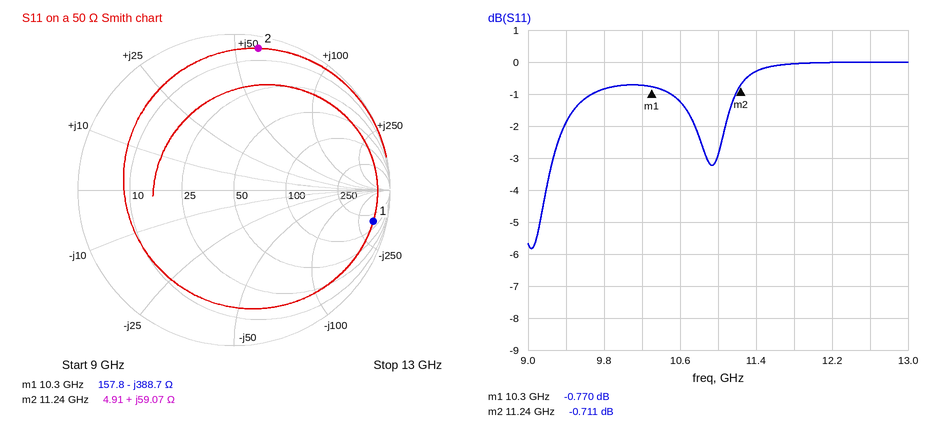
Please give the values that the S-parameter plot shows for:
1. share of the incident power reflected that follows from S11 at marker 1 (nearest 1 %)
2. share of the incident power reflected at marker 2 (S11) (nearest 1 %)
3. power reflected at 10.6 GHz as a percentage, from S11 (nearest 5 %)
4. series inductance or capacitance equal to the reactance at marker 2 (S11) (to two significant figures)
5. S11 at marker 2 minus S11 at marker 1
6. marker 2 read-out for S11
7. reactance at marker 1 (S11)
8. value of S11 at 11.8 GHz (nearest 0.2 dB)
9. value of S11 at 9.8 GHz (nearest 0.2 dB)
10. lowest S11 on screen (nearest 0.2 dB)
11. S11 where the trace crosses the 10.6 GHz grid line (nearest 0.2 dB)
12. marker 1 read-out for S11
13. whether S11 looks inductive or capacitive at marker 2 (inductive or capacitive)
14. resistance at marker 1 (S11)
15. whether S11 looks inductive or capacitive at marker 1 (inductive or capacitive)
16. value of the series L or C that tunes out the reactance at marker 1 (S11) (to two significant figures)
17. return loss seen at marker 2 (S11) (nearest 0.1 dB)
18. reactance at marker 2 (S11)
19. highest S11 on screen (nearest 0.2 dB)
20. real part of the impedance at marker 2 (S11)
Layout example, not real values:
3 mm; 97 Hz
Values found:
84 %; 85 %; 75 %; 840 pH; 0.059 dB; -0.711 dB; -388.7 Ω; 0.0 dB; -0.8 dB; -5.8 dB; -1.2 dB; -0.770 dB; inductive; 157.8 Ω; capacitive; 6.0 nH; 0.7 dB; +59.07 Ω; 0.0 dB; 4.91 Ω
